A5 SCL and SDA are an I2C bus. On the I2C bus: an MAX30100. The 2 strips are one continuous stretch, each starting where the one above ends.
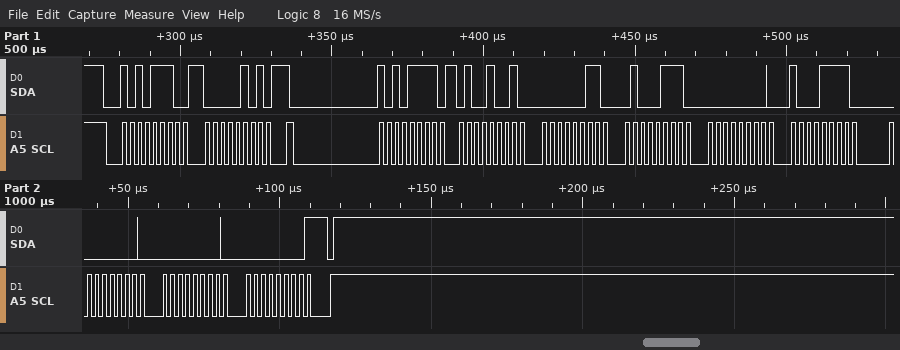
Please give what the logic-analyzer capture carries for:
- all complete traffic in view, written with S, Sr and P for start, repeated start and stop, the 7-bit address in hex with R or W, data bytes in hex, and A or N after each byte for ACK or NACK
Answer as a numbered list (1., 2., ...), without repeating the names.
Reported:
1. S 57W A 05 A Sr 57R A 49 A 03 A 47 A 00 A 8F A 00 A 00 A 00 N P
